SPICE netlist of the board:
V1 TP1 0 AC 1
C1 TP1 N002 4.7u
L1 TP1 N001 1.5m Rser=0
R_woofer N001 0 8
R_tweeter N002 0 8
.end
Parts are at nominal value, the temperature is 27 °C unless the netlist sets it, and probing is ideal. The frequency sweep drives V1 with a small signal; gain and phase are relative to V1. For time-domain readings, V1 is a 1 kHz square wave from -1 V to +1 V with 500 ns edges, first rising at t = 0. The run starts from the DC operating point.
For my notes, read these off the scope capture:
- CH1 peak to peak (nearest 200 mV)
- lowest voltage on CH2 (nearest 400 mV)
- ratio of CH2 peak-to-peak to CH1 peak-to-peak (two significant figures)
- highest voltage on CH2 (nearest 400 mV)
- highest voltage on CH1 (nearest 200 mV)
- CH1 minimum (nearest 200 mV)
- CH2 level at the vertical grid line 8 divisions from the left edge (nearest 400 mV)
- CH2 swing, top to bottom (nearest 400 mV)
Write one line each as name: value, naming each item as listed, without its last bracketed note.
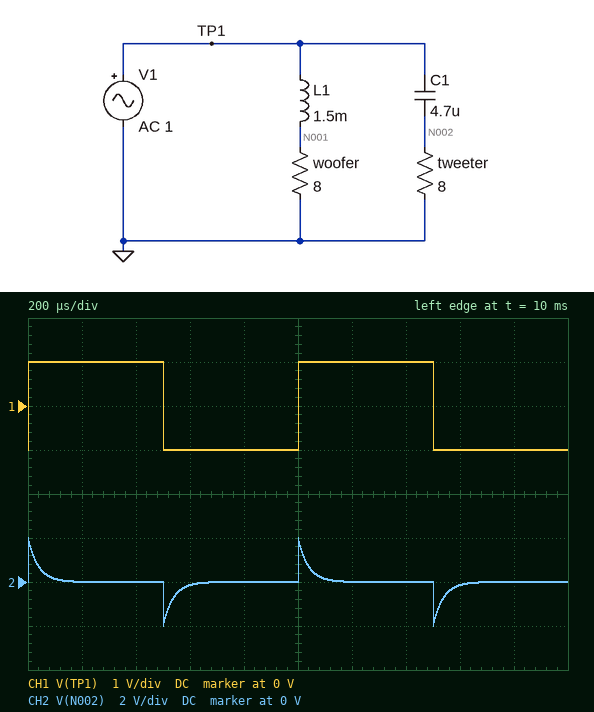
CH1 peak to peak: 2.0 V
lowest voltage on CH2: -2.0 V
ratio of CH2 peak-to-peak to CH1 peak-to-peak: 2.0
highest voltage on CH2: 2.0 V
highest voltage on CH1: 1.0 V
CH1 minimum: -1.0 V
CH2 level at the vertical grid line 8 divisions from the left edge: 0 V
CH2 swing, top to bottom: 4.0 V
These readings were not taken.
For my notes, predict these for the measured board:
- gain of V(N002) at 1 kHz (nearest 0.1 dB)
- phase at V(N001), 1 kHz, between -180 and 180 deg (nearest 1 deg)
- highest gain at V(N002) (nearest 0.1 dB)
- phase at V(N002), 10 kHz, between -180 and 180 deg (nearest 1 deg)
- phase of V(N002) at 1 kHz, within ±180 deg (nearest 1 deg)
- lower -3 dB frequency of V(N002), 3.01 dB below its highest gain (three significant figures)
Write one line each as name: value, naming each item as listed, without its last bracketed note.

gain of V(N002) at 1 kHz: -12.8 dB
phase at V(N001), 1 kHz, between -180 and 180 deg: -50 deg
highest gain at V(N002): 0 dB
phase at V(N002), 10 kHz, between -180 and 180 deg: 23 deg
phase of V(N002) at 1 kHz, within ±180 deg: 77 deg
lower -3 dB frequency of V(N002), 3.01 dB below its highest gain: 4.23 kHz
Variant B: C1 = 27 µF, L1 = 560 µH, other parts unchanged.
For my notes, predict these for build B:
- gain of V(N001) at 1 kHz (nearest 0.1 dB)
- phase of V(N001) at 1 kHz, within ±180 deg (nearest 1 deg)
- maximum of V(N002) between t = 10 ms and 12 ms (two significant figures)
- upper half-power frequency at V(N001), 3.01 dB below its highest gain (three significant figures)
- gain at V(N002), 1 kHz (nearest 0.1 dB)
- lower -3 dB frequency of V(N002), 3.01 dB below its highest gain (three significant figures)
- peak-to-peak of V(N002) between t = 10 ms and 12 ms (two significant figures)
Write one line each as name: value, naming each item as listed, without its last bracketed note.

gain of V(N001) at 1 kHz: -0.8 dB
phase of V(N001) at 1 kHz, within ±180 deg: -24 deg
maximum of V(N002) between t = 10 ms and 12 ms: 1.8 V
upper half-power frequency at V(N001), 3.01 dB below its highest gain: 2.27 kHz
gain at V(N002), 1 kHz: -1.9 dB
lower -3 dB frequency of V(N002), 3.01 dB below its highest gain: 737 Hz
peak-to-peak of V(N002) between t = 10 ms and 12 ms: 3.6 V
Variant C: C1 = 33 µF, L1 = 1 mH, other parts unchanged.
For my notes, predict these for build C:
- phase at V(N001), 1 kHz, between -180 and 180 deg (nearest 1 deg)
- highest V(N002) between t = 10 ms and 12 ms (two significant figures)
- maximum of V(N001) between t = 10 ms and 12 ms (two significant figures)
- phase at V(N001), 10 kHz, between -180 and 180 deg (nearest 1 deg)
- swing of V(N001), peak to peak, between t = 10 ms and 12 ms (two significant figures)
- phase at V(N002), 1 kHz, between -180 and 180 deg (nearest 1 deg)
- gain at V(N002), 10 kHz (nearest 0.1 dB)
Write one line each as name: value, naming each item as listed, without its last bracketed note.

phase at V(N001), 1 kHz, between -180 and 180 deg: -38 deg
highest V(N002) between t = 10 ms and 12 ms: 1.7 V
maximum of V(N001) between t = 10 ms and 12 ms: 960 mV
phase at V(N001), 10 kHz, between -180 and 180 deg: -83 deg
swing of V(N001), peak to peak, between t = 10 ms and 12 ms: 1.9 V
phase at V(N002), 1 kHz, between -180 and 180 deg: 31 deg
gain at V(N002), 10 kHz: 0 dB
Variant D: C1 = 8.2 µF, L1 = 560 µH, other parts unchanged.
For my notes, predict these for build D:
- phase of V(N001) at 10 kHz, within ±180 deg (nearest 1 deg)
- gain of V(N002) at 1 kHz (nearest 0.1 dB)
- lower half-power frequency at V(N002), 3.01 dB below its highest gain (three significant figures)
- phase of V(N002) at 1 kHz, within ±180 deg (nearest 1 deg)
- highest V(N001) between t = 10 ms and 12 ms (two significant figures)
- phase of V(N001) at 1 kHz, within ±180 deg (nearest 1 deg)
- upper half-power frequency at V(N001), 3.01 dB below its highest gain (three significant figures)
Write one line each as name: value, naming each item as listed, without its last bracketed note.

phase of V(N001) at 10 kHz, within ±180 deg: -77 deg
gain of V(N002) at 1 kHz: -8.4 dB
lower half-power frequency at V(N002), 3.01 dB below its highest gain: 2.43 kHz
phase of V(N002) at 1 kHz, within ±180 deg: 68 deg
highest V(N001) between t = 10 ms and 12 ms: 1.0 V
phase of V(N001) at 1 kHz, within ±180 deg: -24 deg
upper half-power frequency at V(N001), 3.01 dB below its highest gain: 2.27 kHz
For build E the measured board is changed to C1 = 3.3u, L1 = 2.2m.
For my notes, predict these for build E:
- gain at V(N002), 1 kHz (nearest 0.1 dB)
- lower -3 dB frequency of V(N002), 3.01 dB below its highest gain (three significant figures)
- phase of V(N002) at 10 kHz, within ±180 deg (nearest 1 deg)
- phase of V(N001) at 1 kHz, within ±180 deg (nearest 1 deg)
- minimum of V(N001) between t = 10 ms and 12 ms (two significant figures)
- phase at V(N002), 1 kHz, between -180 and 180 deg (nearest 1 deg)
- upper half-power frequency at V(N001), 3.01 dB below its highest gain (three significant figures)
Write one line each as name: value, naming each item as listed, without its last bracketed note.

gain at V(N002), 1 kHz: -15.7 dB
lower -3 dB frequency of V(N002), 3.01 dB below its highest gain: 6.03 kHz
phase of V(N002) at 10 kHz, within ±180 deg: 31 deg
phase of V(N001) at 1 kHz, within ±180 deg: -60 deg
minimum of V(N001) between t = 10 ms and 12 ms: -720 mV
phase at V(N002), 1 kHz, between -180 and 180 deg: 81 deg
upper half-power frequency at V(N001), 3.01 dB below its highest gain: 579 Hz
